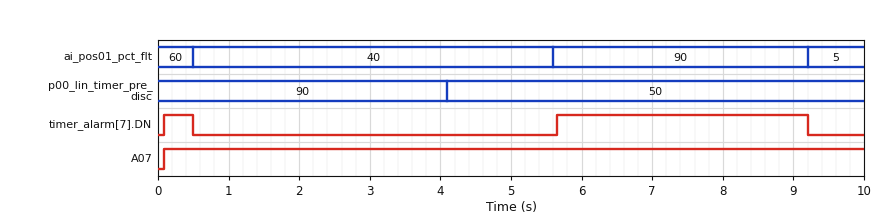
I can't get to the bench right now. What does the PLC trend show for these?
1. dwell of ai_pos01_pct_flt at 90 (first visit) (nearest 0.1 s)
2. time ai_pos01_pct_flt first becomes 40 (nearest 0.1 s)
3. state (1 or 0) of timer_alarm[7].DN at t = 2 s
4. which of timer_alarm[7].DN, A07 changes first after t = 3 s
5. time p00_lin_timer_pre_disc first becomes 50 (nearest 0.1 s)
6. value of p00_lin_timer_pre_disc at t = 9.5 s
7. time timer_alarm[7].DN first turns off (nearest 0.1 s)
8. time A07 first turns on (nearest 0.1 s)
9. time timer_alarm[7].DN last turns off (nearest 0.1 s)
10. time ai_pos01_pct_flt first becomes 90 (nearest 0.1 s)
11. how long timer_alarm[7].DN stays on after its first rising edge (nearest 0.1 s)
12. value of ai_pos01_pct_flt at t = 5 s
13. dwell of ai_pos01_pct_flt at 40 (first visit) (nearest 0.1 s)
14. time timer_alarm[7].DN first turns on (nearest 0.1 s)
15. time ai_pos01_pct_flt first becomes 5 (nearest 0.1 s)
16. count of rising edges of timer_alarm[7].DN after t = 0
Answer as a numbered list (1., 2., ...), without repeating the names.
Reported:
1. 3.6 s
2. 0.5 s
3. 0
4. timer_alarm[7].DN
5. 4.1 s
6. 50
7. 0.5 s
8. 0.1 s
9. 9.2 s
10. 5.6 s
11. 0.4 s
12. 40
13. 5.1 s
14. 0.1 s
15. 9.2 s
16. 2
